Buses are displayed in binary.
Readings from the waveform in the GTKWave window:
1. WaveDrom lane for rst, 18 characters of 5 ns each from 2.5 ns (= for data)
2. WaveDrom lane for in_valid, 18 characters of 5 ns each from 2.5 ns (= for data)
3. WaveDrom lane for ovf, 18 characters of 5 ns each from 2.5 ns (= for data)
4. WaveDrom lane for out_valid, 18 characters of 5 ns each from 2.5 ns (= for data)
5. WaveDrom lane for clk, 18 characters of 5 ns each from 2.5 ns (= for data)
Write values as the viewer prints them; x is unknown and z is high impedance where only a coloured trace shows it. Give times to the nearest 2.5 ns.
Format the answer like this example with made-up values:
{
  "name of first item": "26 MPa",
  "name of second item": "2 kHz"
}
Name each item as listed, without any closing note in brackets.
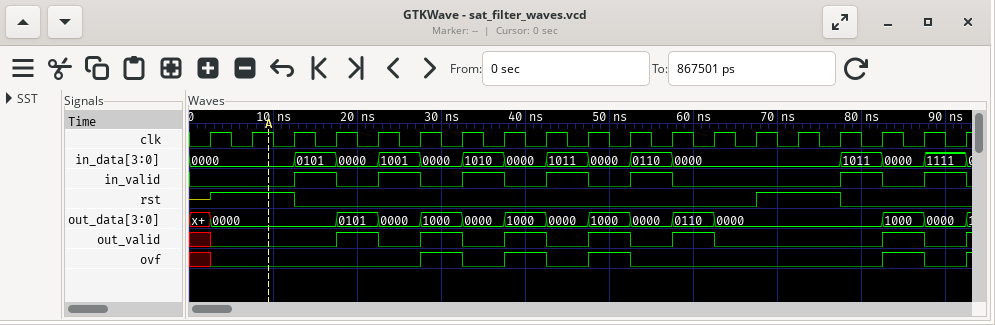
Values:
{
  "WaveDrom lane for rst, 18 characters of 5 ns each from 2.5 ns": "{name: 'rst', wave: '1.0..........1.0..'}",
  "WaveDrom lane for in_valid, 18 characters of 5 ns each from 2.5 ns": "{name: 'in_valid', wave: '0.1010101010...101'}",
  "WaveDrom lane for ovf, 18 characters of 5 ns each from 2.5 ns": "{name: 'ovf', wave: '0....101010.....10'}",
  "WaveDrom lane for out_valid, 18 characters of 5 ns each from 2.5 ns": "{name: 'out_valid', wave: '0..1010101010...10'}",
  "WaveDrom lane for clk, 18 characters of 5 ns each from 2.5 ns": "{name: 'clk', wave: 'p.................'}"
}
